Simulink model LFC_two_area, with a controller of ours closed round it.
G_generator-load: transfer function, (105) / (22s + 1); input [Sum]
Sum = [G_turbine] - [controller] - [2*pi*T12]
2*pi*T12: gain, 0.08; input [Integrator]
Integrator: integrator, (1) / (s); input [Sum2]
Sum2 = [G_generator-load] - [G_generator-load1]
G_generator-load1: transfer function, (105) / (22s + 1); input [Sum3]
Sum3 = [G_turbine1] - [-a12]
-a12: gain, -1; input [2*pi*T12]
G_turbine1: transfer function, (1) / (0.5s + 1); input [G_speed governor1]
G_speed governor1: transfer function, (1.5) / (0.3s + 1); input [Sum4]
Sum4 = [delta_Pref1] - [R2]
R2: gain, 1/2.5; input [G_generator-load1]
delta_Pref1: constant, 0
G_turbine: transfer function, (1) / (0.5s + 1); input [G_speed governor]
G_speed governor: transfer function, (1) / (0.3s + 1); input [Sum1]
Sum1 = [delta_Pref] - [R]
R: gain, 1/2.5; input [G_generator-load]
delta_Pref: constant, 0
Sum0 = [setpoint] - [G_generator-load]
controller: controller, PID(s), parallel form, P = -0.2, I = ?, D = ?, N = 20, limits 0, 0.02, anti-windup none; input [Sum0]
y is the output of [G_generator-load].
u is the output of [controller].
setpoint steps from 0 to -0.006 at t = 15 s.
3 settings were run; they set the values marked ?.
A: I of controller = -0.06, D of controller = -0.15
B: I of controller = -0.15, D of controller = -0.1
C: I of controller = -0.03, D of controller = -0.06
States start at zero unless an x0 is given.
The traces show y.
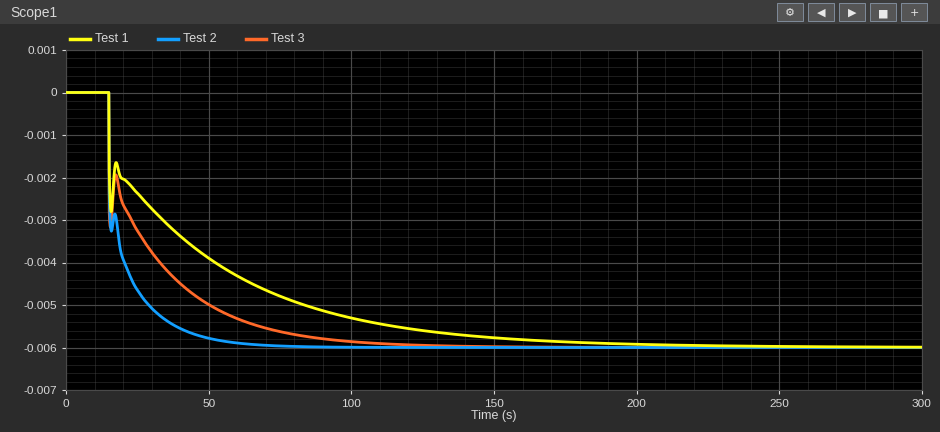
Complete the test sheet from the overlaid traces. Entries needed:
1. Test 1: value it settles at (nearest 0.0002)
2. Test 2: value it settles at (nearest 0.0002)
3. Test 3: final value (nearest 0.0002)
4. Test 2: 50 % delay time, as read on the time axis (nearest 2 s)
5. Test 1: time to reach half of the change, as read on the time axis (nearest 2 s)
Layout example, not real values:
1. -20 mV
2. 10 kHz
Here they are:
1. -0.0060
2. -0.0060
3. -0.0060
4. 16 s
5. 34 s
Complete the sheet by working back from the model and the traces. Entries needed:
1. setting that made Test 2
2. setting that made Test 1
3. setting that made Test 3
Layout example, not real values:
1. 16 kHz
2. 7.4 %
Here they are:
1. B
2. C
3. A
